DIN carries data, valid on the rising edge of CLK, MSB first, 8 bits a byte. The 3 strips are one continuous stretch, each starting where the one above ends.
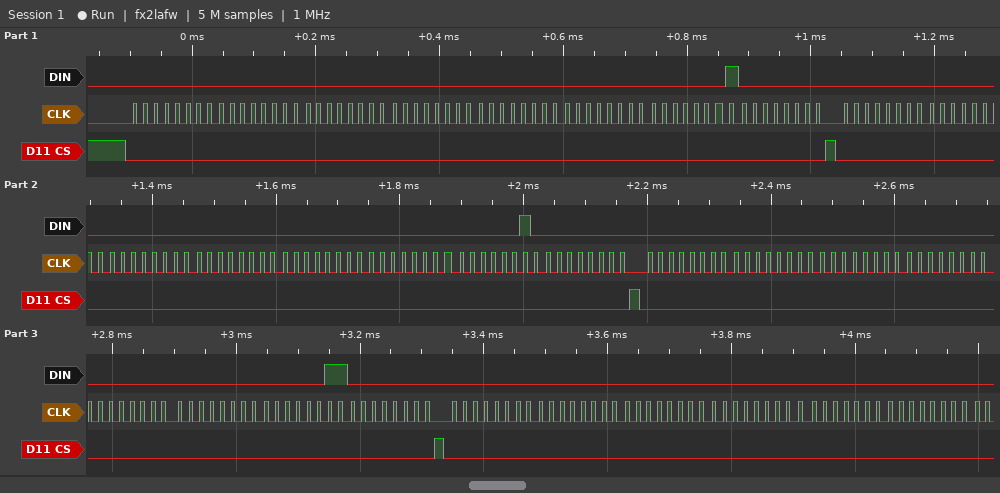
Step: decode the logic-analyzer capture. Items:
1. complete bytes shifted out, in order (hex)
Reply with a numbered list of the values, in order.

1. 00 00 00 00 00 00 01 00 00 00 00 00 00 00 02 00 00 00 00 00 00 00 03 00 00 00 00 00 00 00
